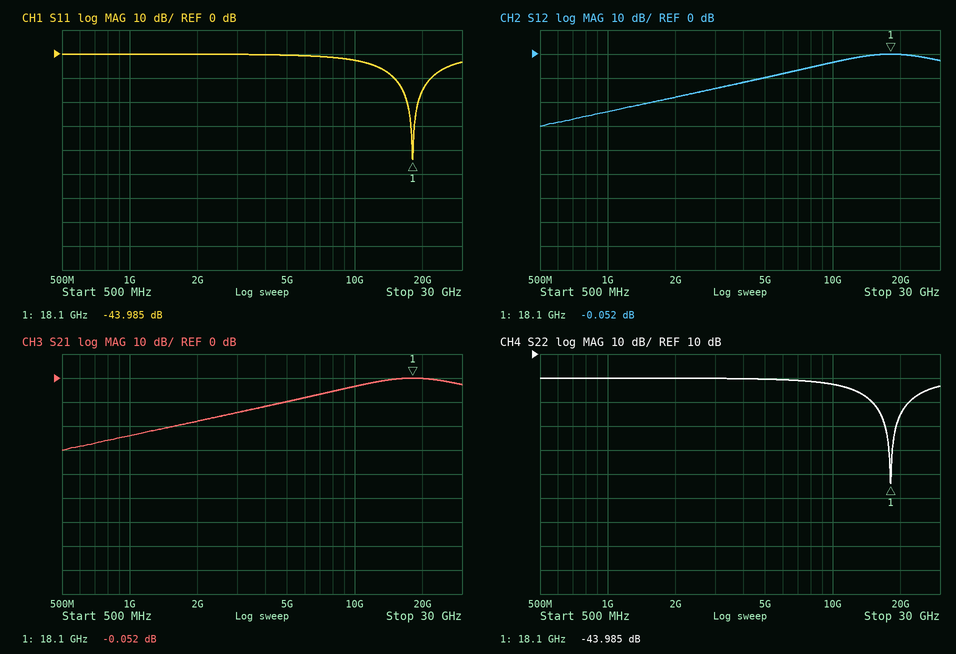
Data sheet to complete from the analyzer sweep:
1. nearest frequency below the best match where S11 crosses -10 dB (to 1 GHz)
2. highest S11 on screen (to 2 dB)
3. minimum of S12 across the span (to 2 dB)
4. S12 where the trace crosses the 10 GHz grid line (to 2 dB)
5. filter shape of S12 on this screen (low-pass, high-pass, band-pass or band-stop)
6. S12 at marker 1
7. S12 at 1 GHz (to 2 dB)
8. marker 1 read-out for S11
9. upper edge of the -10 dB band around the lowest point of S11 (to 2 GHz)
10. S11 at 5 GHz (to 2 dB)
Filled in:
15 GHz
0 dB
-30 dB
-4 dB
high-pass
-0.052 dB
-24 dB
-43.985 dB
22 GHz
0 dB
